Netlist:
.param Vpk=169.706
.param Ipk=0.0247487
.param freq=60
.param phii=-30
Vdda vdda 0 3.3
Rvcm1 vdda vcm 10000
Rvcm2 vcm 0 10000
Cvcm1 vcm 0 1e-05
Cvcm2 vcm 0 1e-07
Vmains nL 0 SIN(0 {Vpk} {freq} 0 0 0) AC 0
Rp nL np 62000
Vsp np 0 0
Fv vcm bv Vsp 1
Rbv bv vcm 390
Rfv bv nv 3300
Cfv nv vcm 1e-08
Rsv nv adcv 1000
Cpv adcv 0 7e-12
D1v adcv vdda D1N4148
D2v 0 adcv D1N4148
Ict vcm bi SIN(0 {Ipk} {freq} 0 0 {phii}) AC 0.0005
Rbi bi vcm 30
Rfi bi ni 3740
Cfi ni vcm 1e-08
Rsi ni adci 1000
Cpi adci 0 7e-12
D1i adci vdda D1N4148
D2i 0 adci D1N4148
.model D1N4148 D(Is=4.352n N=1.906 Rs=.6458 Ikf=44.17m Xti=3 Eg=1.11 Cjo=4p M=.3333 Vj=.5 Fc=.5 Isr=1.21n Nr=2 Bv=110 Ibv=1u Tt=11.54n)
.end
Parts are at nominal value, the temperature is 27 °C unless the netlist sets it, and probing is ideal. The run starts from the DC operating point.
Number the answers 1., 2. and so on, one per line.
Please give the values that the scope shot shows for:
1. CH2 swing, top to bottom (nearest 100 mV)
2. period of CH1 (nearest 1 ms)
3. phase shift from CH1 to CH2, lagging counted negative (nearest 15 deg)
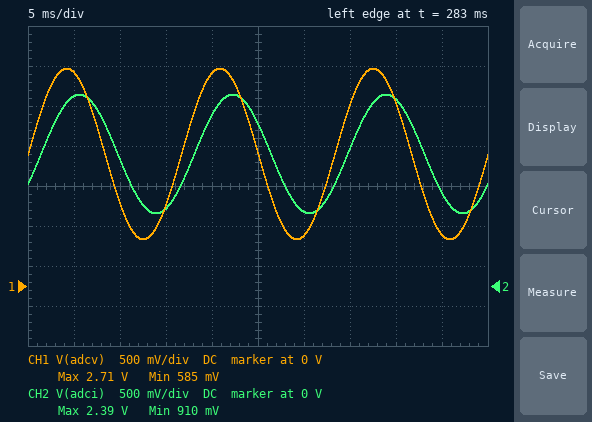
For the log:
1. 1.5 V
2. 17 ms
3. -30 deg
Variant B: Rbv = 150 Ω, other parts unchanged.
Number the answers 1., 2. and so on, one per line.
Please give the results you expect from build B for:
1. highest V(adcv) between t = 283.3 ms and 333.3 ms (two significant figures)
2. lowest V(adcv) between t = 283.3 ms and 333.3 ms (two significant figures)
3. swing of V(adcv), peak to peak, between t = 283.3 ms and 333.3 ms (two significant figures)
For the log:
1. 2.1 V
2. 1.2 V
3. 820 mV
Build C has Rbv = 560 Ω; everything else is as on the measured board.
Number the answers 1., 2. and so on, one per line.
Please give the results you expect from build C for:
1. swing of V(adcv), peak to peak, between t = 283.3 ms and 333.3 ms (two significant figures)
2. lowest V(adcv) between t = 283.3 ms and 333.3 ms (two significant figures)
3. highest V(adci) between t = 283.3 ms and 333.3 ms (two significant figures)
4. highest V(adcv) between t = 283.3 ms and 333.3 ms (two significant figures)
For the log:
1. 3.1 V
2. 120 mV
3. 2.4 V
4. 3.2 V
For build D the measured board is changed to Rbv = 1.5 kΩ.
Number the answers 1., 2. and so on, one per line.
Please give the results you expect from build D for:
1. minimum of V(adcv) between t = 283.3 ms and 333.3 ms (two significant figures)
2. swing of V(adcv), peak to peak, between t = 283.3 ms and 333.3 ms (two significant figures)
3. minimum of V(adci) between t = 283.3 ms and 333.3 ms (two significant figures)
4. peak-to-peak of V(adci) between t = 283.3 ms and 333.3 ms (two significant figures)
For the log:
1. -550 mV
2. 4.4 V
3. 950 mV
4. 1.4 V
